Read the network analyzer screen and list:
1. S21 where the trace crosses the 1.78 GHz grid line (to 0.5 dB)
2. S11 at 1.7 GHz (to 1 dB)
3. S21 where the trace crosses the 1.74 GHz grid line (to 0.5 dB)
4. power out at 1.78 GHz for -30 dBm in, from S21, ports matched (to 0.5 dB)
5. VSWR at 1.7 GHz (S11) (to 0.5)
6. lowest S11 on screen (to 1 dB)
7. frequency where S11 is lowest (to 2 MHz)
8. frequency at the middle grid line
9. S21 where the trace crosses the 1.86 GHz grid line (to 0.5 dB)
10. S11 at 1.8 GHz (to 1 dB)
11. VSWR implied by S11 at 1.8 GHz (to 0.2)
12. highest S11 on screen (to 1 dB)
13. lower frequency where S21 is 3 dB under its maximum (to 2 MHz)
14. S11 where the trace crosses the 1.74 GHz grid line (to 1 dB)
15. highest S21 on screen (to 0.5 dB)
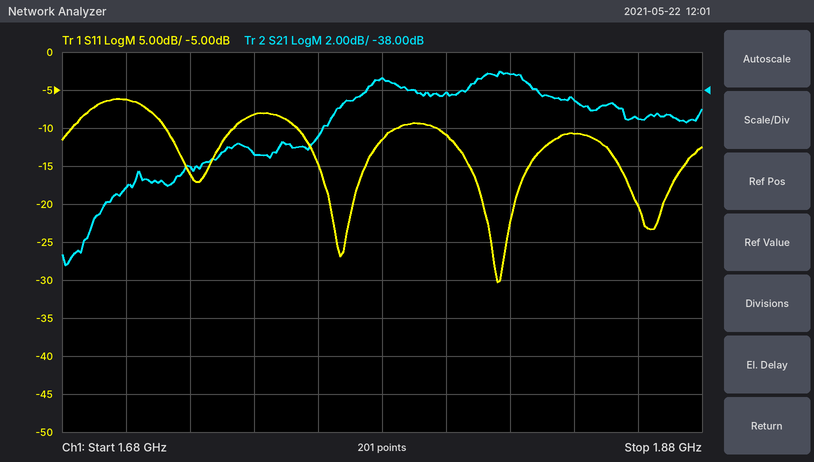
-37.5 dB
-6 dB
-41.5 dB
-67.5 dBm
3.0
-30 dB
1.816 GHz
1.78 GHz
-39.5 dB
-11 dB
1.8
-6 dB
1.762 GHz
-8 dB
-37.0 dB
